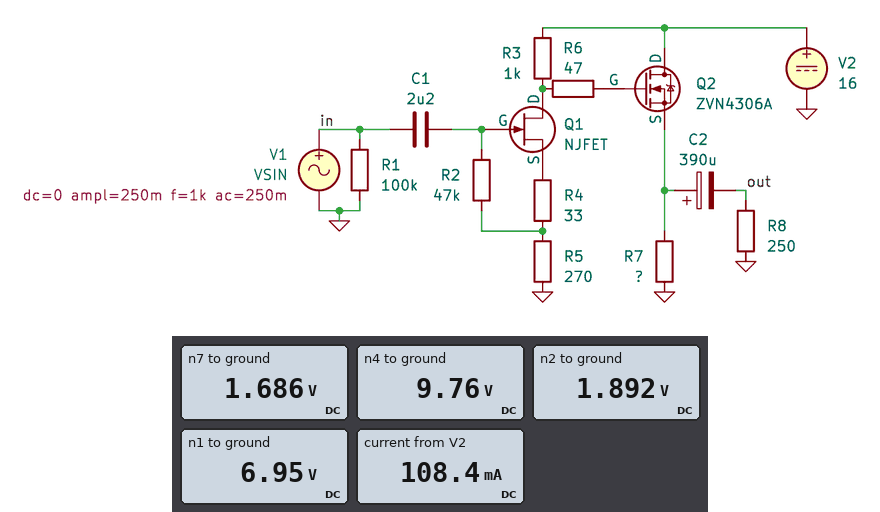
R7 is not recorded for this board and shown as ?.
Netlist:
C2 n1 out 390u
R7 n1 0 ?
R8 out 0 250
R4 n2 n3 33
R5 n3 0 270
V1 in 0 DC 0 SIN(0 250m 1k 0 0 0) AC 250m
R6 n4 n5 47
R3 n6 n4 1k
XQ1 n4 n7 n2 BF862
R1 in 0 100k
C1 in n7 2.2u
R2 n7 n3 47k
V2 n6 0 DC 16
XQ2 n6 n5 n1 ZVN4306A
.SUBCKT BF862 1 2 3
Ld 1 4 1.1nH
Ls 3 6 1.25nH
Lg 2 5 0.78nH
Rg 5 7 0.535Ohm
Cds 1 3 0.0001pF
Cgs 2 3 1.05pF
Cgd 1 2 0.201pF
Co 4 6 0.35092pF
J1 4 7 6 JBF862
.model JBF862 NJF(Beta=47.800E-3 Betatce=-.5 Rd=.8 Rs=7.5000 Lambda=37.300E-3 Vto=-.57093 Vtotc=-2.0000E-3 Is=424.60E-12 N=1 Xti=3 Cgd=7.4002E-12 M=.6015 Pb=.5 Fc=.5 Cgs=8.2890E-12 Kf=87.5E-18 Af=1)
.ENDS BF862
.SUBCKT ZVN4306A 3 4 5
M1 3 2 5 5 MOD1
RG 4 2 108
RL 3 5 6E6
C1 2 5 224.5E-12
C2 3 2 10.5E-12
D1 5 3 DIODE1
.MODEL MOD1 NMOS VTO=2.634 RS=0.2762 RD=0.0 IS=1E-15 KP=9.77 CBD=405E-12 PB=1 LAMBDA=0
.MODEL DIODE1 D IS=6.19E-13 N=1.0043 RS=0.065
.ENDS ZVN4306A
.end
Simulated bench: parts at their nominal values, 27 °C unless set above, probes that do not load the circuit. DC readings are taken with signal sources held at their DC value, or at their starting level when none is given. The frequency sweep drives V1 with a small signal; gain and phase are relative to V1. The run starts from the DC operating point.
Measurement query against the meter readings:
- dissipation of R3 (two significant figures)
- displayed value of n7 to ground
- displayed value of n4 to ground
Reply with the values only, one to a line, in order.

39 mW
1.686 V
9.76 V
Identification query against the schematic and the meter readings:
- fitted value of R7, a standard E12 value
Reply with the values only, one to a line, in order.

68 Ω
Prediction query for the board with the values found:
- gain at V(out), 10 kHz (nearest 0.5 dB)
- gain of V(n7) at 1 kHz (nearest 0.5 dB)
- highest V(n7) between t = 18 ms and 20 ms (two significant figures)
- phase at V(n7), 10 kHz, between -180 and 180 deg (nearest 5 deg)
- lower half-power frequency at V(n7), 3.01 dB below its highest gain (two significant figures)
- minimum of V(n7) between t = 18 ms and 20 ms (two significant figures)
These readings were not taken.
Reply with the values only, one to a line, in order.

9.0 dB
0 dB
1.9 V
0 deg
320 mHz
1.4 V
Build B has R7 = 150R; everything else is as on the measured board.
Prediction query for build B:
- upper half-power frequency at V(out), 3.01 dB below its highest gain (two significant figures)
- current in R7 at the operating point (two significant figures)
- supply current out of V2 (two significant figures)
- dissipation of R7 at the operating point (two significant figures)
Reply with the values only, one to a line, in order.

11 MHz
47 mA
53 mA
330 mW
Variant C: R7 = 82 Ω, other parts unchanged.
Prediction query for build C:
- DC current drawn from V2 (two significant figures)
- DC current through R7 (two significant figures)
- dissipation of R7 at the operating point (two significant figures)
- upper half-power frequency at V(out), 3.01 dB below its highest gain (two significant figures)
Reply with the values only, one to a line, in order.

91 mA
85 mA
590 mW
9.8 MHz
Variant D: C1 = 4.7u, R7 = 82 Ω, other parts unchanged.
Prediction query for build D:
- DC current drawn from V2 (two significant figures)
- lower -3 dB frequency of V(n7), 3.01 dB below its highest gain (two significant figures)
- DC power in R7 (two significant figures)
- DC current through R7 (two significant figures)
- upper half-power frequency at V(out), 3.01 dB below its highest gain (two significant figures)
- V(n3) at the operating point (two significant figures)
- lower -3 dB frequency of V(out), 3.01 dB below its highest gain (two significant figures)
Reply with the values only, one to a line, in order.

91 mA
150 mHz
590 mW
85 mA
9.8 MHz
1.7 V
1.6 Hz
